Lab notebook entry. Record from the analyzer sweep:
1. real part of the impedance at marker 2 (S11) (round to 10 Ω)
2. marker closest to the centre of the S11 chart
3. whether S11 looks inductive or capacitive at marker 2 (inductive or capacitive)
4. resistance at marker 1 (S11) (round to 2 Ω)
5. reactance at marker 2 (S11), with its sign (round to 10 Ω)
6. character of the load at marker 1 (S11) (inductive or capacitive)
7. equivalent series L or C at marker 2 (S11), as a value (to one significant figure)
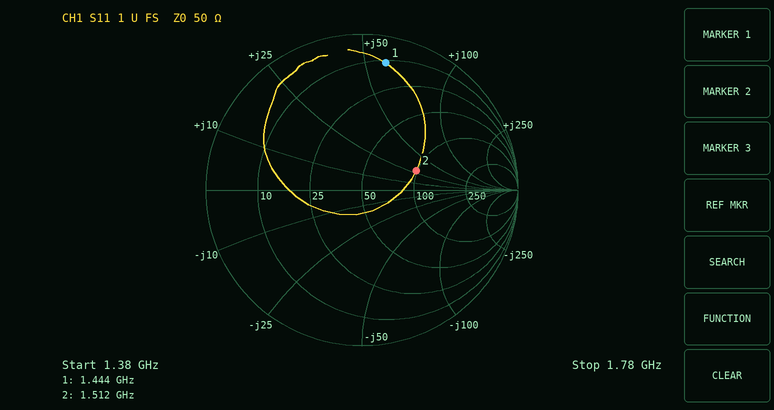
100 Ω
marker 2
inductive
12 Ω
+30 Ω
inductive
3 nH
